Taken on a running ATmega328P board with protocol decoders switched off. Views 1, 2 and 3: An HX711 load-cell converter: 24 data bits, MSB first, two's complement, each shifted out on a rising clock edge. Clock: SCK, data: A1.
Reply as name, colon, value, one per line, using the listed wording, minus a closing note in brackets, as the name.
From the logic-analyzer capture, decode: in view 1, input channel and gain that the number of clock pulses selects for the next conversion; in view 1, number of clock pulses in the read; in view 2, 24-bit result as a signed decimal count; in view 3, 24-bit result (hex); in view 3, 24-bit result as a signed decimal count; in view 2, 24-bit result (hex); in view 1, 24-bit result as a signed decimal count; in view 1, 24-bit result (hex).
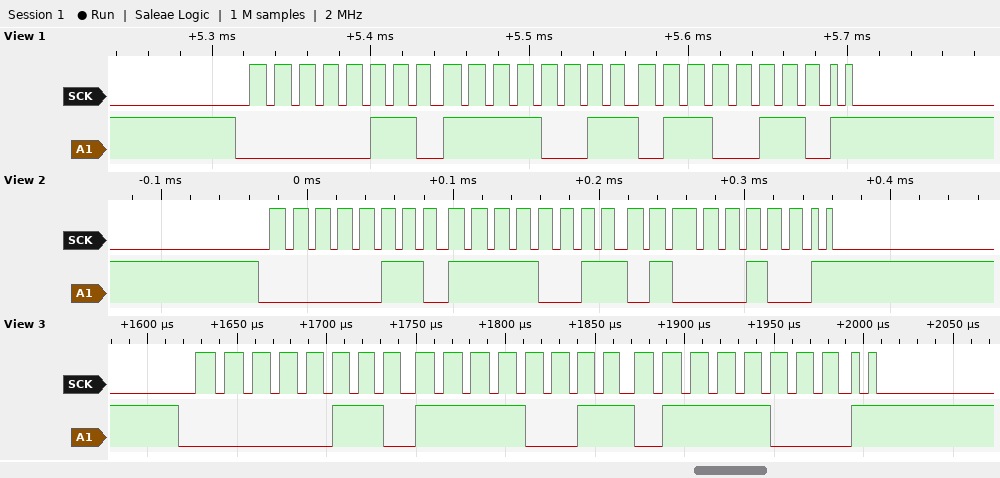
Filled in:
in view 1, input channel and gain that the number of clock pulses selects for the next conversion: channel B, gain 32
in view 1, number of clock pulses in the read: 26
in view 2, 24-bit result as a signed decimal count: 455492
in view 3, 24-bit result: 0x06F378
in view 3, 24-bit result as a signed decimal count: 455544
in view 2, 24-bit result: 0x06F344
in view 1, 24-bit result as a signed decimal count: 455526
in view 1, 24-bit result: 0x06F366
